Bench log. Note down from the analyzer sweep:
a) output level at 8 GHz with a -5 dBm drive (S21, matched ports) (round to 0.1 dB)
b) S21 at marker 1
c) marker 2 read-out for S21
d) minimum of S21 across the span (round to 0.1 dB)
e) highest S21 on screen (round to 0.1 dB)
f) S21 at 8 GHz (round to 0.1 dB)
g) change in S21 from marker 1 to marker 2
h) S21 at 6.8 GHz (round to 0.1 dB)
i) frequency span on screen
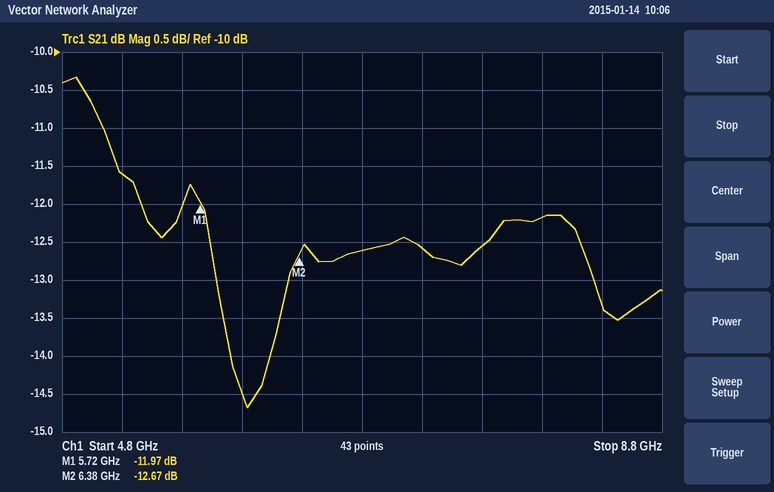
-17.2 dBm
-11.97 dB
-12.67 dB
-14.7 dB
-10.3 dB
-12.2 dB
-0.70 dB
-12.6 dB
4 GHz
